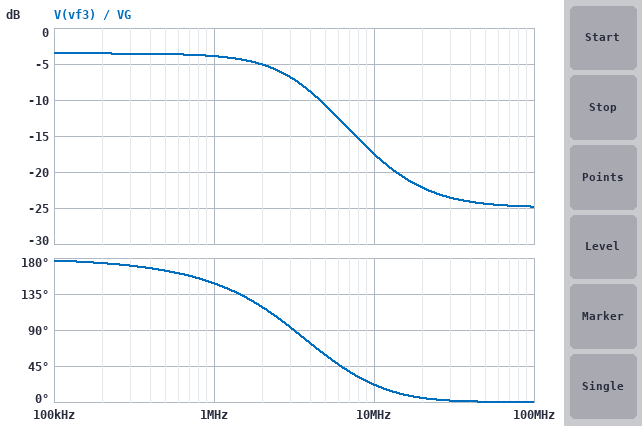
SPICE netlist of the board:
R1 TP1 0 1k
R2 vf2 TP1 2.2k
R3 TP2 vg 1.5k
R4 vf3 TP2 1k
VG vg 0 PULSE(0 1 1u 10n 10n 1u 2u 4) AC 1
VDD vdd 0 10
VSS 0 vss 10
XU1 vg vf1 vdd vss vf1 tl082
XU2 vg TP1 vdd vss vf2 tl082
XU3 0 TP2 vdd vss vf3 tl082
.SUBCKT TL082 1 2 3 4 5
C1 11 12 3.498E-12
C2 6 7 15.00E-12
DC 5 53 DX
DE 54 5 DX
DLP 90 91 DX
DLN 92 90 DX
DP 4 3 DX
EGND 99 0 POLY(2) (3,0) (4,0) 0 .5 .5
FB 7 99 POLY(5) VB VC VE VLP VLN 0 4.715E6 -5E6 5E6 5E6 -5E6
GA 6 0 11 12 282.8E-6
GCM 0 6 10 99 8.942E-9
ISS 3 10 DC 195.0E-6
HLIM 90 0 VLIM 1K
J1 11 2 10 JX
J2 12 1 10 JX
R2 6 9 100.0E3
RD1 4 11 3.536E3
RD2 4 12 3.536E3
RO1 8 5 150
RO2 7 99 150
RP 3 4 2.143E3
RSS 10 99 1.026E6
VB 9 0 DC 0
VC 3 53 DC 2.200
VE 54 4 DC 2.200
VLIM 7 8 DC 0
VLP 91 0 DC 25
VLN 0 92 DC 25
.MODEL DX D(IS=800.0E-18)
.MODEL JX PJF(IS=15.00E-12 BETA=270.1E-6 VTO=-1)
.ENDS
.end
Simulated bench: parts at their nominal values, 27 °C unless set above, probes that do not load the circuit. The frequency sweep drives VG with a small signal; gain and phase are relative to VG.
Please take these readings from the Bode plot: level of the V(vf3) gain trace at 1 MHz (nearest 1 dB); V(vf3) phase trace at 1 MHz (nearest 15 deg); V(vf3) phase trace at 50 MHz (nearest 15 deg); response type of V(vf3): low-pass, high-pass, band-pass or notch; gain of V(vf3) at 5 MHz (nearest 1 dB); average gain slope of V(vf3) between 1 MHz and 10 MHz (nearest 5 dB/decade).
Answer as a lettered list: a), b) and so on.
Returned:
a) -4 dB
b) 150 deg
c) 0 deg
d) low-pass
e) -11 dB
f) -15 dB/decade
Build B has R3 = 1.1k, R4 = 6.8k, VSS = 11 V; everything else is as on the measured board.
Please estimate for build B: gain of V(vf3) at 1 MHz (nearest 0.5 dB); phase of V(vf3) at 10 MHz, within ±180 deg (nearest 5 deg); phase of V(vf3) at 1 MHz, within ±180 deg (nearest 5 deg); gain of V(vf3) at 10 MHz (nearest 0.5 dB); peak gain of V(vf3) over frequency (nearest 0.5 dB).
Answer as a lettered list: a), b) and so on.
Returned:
a) 9.0 dB
b) 30 deg
c) 105 deg
d) -15.0 dB
e) 16.0 dB
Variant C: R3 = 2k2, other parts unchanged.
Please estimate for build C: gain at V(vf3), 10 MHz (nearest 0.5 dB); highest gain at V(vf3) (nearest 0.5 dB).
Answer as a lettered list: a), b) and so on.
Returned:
a) -19.5 dB
b) -7.0 dB
